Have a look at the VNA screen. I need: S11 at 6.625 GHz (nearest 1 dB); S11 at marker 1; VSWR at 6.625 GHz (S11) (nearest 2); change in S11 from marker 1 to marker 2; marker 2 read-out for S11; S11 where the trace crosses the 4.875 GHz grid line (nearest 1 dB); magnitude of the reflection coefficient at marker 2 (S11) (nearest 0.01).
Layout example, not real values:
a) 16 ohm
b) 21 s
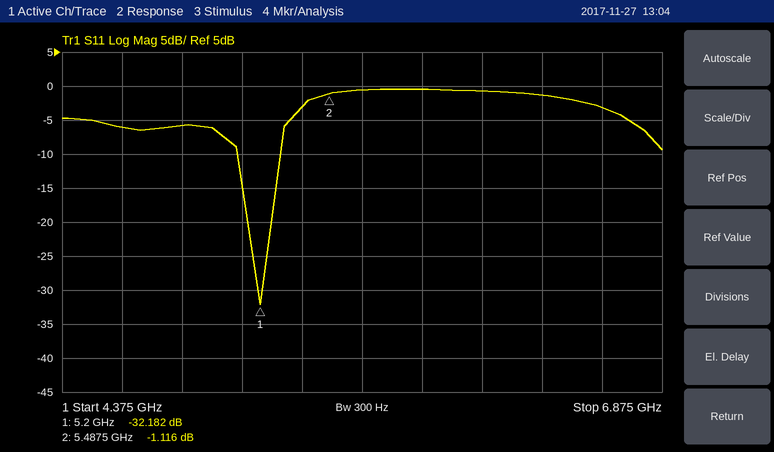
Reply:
a) -3 dB
b) -32.182 dB
c) 6
d) 31.066 dB
e) -1.116 dB
f) -6 dB
g) 0.88
